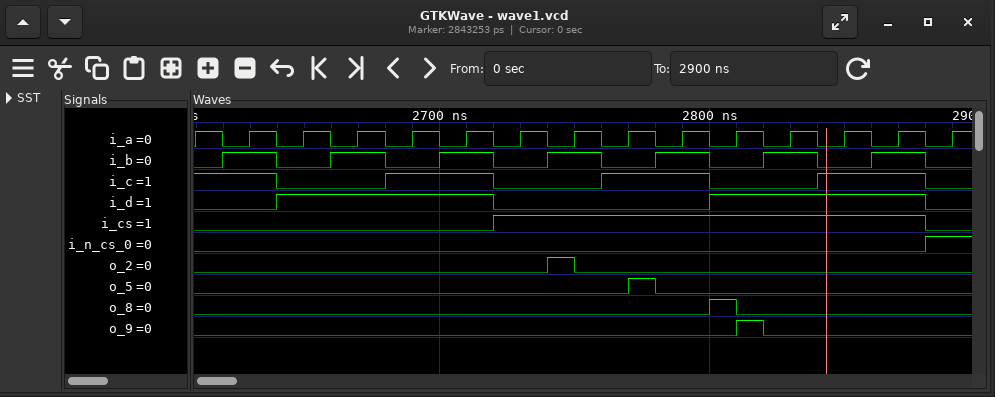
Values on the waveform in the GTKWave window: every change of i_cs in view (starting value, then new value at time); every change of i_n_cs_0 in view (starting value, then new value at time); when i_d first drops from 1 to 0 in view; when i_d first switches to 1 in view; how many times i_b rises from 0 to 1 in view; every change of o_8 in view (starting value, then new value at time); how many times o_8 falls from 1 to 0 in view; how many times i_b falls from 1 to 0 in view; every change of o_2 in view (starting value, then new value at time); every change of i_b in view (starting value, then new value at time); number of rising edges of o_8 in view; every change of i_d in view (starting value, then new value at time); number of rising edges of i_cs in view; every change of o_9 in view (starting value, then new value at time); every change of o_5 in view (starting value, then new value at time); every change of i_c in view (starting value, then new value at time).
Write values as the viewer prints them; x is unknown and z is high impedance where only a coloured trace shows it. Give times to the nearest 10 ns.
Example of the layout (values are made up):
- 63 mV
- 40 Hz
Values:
- 0, 1 at 2720 ns, 0 at 2880 ns
- 0, 1 at 2880 ns
- 2720 ns
- 2640 ns
- 7
- 0, 1 at 2800 ns, 0 at 2810 ns
- 1
- 7
- 0, 1 at 2740 ns, 0 at 2750 ns
- 0, 1 at 2620 ns, 0 at 2640 ns, 1 at 2660 ns, 0 at 2680 ns, 1 at 2700 ns, 0 at 2720 ns, 1 at 2740 ns, 0 at 2760 ns, 1 at 2780 ns, 0 at 2800 ns, 1 at 2820 ns, 0 at 2840 ns, 1 at 2860 ns, 0 at 2880 ns
- 1
- 0, 1 at 2640 ns, 0 at 2720 ns, 1 at 2800 ns, 0 at 2880 ns
- 1
- 0, 1 at 2810 ns, 0 at 2820 ns
- 0, 1 at 2770 ns, 0 at 2780 ns
- 1, 0 at 2640 ns, 1 at 2680 ns, 0 at 2720 ns, 1 at 2760 ns, 0 at 2800 ns, 1 at 2840 ns, 0 at 2880 ns
